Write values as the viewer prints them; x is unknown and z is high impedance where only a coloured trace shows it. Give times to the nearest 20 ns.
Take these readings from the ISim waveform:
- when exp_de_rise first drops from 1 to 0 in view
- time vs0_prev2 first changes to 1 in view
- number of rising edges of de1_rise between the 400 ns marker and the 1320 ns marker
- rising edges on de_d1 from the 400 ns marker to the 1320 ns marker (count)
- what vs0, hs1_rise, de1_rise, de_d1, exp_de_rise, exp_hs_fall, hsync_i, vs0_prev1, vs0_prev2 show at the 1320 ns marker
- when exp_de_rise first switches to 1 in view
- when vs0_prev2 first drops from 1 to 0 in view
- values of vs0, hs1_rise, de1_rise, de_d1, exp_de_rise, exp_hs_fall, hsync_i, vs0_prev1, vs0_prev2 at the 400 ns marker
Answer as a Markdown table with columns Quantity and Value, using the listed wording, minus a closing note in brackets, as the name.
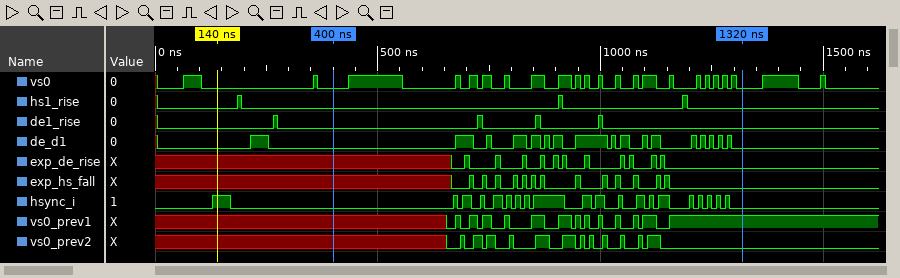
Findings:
| Quantity | Value |
|---|---|
| when exp_de_rise first drops from 1 to 0 in view | 700 ns |
| time vs0_prev2 first changes to 1 in view | 680 ns |
| number of rising edges of de1_rise between the 400 ns marker and the 1320 ns marker | 3 |
| rising edges on de_d1 from the 400 ns marker to the 1320 ns marker | 16 |
| what vs0, hs1_rise, de1_rise, de_d1, exp_de_rise, exp_hs_fall, hsync_i, vs0_prev1, vs0_prev2 show at the 1320 ns marker | vs0=0, hs1_rise=0, de1_rise=0, de_d1=0, exp_de_rise=0, exp_hs_fall=0, hsync_i=0, vs0_prev1=1, vs0_prev2=0 |
| when exp_de_rise first switches to 1 in view | 700 ns |
| when vs0_prev2 first drops from 1 to 0 in view | 700 ns |
| values of vs0, hs1_rise, de1_rise, de_d1, exp_de_rise, exp_hs_fall, hsync_i, vs0_prev1, vs0_prev2 at the 400 ns marker | vs0=0, hs1_rise=0, de1_rise=0, de_d1=0, exp_de_rise=x, exp_hs_fall=x, hsync_i=0, vs0_prev1=x, vs0_prev2=x |
